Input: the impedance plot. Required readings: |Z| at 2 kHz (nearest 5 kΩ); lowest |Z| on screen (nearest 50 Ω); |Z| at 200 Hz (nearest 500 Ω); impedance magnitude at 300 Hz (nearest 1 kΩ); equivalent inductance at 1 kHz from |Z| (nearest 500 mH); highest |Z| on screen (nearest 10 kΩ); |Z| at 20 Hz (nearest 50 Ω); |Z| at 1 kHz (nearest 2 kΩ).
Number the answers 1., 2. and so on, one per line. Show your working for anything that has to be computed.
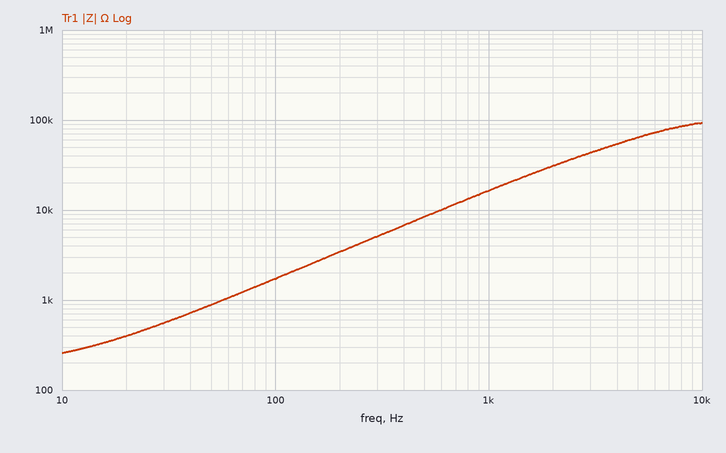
1. 30 kΩ
2. 250 Ω
3. 3.5 kΩ
4. 5 kΩ
5. L = 16 kΩ/(2π × 1 kHz) ≈ 2.5 H
6. 90 kΩ
7. 400 Ω
8. 16 kΩ
